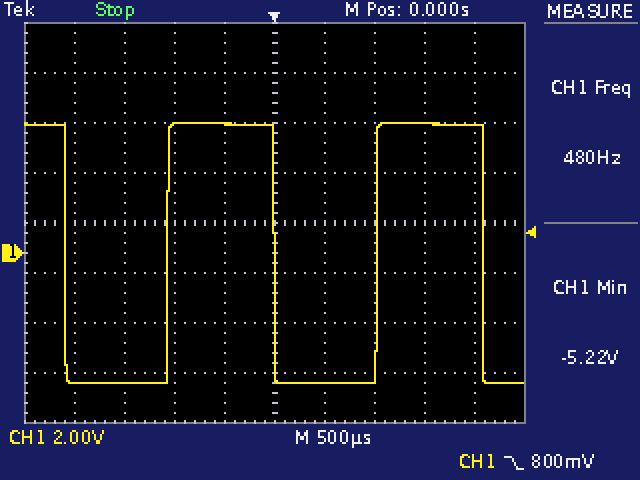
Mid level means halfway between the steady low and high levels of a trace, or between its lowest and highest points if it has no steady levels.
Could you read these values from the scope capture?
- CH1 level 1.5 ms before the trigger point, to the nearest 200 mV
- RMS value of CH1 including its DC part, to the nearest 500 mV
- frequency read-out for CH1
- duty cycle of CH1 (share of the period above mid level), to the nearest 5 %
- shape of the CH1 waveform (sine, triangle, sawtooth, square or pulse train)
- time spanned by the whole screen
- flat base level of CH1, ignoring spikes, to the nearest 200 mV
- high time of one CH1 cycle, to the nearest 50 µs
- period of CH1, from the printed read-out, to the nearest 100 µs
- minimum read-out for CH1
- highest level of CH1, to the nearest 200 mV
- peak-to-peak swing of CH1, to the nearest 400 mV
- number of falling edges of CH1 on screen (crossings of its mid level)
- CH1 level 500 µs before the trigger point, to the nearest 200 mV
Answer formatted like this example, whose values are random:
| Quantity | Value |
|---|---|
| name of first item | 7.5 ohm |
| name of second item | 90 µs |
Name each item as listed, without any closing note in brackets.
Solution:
| Quantity | Value |
|---|---|
| CH1 level 1.5 ms before the trigger point, to the nearest 200 mV | -5.2 V |
| RMS value of CH1 including its DC part, to the nearest 500 mV | 5.0 V |
| frequency read-out for CH1 | 480 Hz |
| duty cycle of CH1 (share of the period above mid level), to the nearest 5 % | 50 % |
| shape of the CH1 waveform | square |
| time spanned by the whole screen | 5 ms |
| flat base level of CH1, ignoring spikes, to the nearest 200 mV | -5.2 V |
| high time of one CH1 cycle, to the nearest 50 µs | 1.05 ms |
| period of CH1, from the printed read-out, to the nearest 100 µs | 2.1 ms |
| minimum read-out for CH1 | -5.22 V |
| highest level of CH1, to the nearest 200 mV | 5.2 V |
| peak-to-peak swing of CH1, to the nearest 400 mV | 10.4 V |
| number of falling edges of CH1 on screen | 3 |
| CH1 level 500 µs before the trigger point, to the nearest 200 mV | 5.2 V |
